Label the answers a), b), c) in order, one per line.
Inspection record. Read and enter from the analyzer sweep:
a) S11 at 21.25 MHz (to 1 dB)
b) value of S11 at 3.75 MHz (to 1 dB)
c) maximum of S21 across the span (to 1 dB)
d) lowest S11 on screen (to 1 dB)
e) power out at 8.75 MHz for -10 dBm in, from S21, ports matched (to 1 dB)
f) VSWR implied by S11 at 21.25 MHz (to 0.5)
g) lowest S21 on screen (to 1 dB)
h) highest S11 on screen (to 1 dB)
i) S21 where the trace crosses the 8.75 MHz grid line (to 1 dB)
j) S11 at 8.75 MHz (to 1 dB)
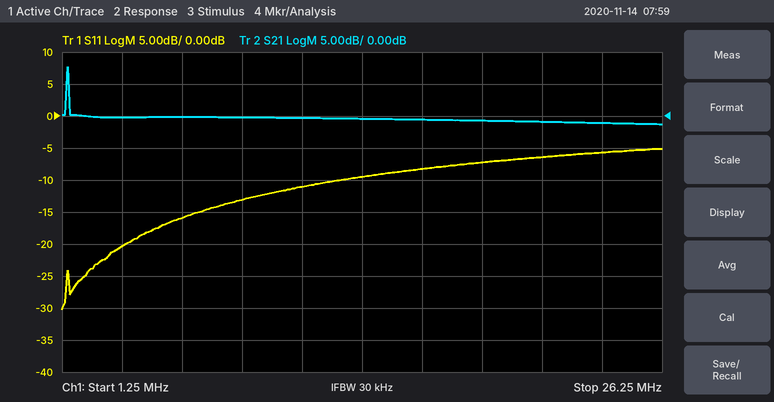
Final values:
a) -6 dB
b) -20 dB
c) 8 dB
d) -30 dB
e) -10 dBm
f) 3.0
g) -1 dB
h) -5 dB
i) 0 dB
j) -13 dB
